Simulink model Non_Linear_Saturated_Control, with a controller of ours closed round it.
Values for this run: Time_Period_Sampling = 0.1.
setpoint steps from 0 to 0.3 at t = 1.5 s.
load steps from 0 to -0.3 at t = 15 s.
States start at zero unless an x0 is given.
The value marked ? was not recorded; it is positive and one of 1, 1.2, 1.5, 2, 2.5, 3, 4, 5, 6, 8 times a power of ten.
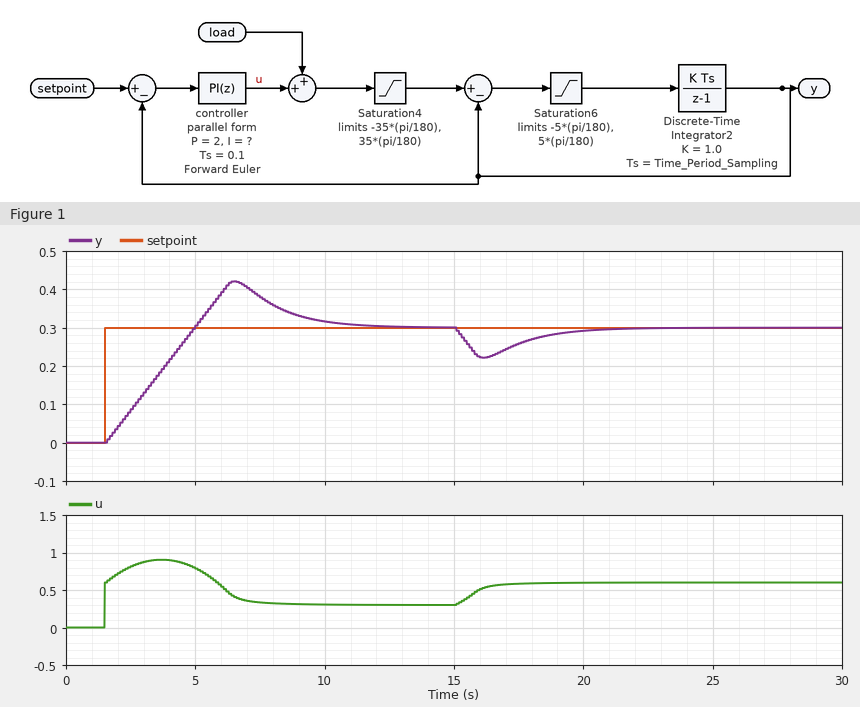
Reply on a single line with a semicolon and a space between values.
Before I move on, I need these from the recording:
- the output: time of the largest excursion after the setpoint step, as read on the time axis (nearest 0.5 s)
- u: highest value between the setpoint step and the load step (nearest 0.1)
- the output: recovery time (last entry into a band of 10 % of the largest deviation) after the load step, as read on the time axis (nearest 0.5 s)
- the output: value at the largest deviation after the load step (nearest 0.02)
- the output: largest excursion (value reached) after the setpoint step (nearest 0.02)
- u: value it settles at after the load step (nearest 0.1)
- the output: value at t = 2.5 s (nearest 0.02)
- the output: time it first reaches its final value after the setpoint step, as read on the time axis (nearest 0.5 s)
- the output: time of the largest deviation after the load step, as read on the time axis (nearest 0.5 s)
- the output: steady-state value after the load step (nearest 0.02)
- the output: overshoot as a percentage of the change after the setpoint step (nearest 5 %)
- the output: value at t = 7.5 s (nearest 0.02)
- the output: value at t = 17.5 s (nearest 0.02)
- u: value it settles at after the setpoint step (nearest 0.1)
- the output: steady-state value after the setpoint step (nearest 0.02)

6.5 s; 0.9; 20.0 s; 0.22; 0.42; 0.6; 0.08; 5.0 s; 16.0 s; 0.30; 40 %; 0.38; 0.26; 0.3; 0.30
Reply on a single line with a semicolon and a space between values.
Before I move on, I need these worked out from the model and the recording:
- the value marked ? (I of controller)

1.5
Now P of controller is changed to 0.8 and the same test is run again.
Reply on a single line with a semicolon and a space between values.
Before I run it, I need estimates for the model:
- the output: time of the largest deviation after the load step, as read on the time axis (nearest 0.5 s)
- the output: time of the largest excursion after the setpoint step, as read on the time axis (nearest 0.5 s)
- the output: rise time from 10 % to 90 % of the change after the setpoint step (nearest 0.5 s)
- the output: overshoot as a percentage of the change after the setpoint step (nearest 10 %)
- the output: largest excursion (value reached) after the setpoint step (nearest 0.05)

16.5 s; 7.0 s; 2.5 s; 50 %; 0.45
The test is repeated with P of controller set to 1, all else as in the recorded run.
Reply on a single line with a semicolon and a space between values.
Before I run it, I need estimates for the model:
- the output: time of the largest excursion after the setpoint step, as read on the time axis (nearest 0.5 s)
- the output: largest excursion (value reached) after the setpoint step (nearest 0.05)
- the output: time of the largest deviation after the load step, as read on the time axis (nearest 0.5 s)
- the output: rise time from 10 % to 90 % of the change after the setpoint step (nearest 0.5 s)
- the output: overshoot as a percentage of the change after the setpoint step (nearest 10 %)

7.0 s; 0.45; 16.5 s; 2.5 s; 50 %
